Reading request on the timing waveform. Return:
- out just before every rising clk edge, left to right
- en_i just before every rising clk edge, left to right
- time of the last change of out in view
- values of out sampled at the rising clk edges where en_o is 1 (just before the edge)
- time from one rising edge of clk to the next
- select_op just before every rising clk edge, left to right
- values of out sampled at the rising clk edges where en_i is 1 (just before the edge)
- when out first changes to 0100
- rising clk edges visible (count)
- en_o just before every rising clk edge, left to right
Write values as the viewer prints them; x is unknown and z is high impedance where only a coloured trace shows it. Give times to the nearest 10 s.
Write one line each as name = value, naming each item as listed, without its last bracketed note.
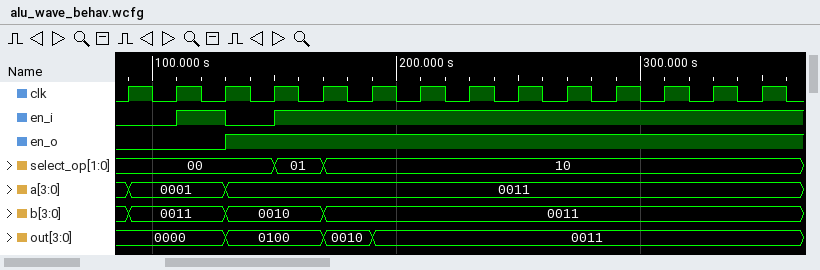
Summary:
out just before every rising clk edge, left to right = 0000, 0000, 0000, 0100, 0100, 0010, 0011, 0011, 0011, 0011, 0011, 0011, 0011, 0011
en_i just before every rising clk edge, left to right = 0 0 1 0 1 1 1 1 1 1 1 1 1 1
time of the last change of out in view = 190 s
values of out sampled at the rising clk edges where en_o is 1 = 0100, 0100, 0010, 0011, 0011, 0011, 0011, 0011, 0011, 0011, 0011
time from one rising edge of clk to the next = 20 s
select_op just before every rising clk edge, left to right = 00, 00, 00, 00, 01, 10, 10, 10, 10, 10, 10, 10, 10, 10
values of out sampled at the rising clk edges where en_i is 1 = 0000, 0100, 0010, 0011, 0011, 0011, 0011, 0011, 0011, 0011, 0011
when out first changes to 0100 = 130 s
rising clk edges visible = 14
en_o just before every rising clk edge, left to right = 0 0 0 1 1 1 1 1 1 1 1 1 1 1
